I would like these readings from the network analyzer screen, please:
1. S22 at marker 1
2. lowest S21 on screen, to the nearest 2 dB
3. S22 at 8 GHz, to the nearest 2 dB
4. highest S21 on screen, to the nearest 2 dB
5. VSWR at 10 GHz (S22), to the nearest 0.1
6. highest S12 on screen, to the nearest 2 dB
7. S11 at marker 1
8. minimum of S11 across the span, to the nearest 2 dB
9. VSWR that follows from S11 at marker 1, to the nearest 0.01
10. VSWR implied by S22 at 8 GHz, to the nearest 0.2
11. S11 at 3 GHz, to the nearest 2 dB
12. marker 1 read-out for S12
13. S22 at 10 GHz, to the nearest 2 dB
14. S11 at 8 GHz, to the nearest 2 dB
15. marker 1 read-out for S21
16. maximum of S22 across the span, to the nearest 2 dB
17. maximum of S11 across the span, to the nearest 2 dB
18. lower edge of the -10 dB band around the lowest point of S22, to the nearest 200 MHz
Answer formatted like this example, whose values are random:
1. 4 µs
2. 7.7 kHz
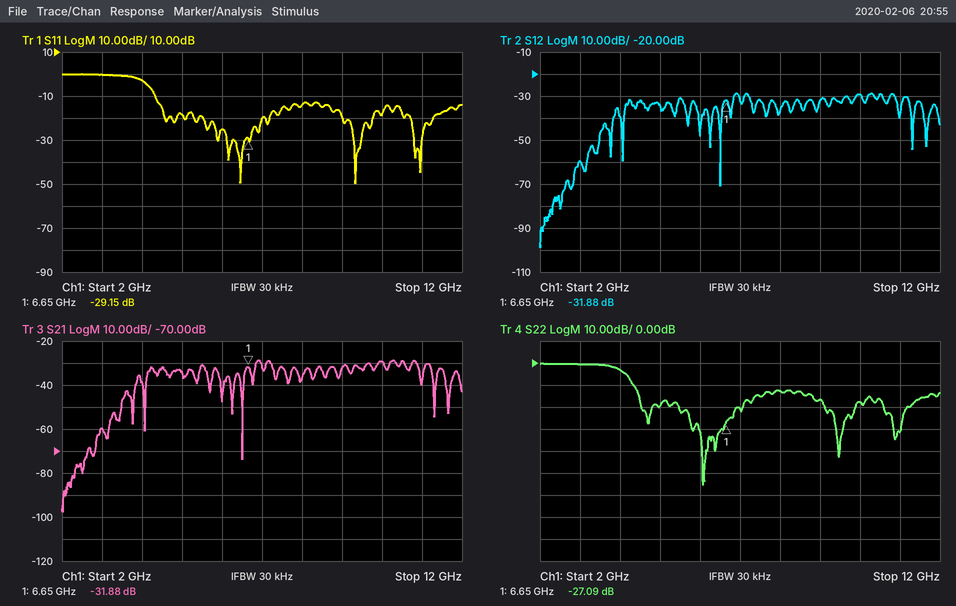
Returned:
1. -27.09 dB
2. -98 dB
3. -12 dB
4. -28 dB
5. 1.3
6. -28 dB
7. -29.15 dB
8. -50 dB
9. 1.07
10. 1.6
11. 0 dB
12. -31.88 dB
13. -18 dB
14. -14 dB
15. -31.88 dB
16. 0 dB
17. 0 dB
18. 4.4 GHz
